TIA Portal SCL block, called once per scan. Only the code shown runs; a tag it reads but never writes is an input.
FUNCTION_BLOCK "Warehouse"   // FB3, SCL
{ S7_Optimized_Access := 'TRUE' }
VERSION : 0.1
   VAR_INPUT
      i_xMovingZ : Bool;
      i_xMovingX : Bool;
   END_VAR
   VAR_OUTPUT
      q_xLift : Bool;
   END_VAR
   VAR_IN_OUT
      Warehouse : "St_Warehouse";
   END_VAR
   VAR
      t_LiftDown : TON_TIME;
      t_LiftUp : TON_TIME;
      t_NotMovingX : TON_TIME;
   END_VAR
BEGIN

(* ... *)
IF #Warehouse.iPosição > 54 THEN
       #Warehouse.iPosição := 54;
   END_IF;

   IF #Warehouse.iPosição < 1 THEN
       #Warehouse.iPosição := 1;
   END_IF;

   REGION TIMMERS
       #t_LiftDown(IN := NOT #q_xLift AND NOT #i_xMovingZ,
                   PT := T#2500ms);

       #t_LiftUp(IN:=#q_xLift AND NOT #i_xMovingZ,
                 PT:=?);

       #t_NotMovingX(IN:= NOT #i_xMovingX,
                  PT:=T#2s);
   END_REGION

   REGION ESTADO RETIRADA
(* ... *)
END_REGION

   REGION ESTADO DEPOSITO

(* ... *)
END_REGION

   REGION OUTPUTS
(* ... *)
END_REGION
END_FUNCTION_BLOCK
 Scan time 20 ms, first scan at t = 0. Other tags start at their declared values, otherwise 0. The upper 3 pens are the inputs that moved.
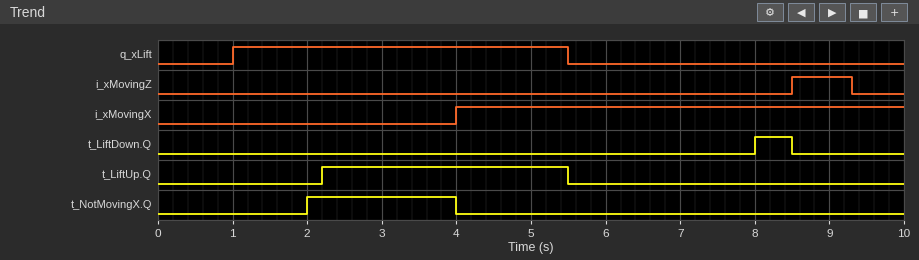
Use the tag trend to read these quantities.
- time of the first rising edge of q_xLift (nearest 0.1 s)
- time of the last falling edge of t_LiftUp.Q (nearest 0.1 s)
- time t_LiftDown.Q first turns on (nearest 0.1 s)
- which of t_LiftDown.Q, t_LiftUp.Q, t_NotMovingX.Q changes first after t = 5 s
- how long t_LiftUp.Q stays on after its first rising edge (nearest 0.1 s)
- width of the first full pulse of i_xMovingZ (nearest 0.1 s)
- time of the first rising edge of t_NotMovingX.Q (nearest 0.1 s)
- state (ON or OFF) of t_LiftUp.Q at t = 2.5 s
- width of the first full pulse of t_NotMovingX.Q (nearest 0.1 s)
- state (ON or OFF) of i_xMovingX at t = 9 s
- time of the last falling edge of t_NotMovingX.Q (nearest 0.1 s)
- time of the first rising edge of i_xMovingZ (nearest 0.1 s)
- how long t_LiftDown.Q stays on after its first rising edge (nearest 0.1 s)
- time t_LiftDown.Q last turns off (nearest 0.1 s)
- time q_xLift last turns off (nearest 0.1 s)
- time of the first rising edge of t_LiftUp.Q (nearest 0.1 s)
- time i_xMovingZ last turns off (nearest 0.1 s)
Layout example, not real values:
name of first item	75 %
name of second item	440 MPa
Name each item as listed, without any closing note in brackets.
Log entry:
time of the first rising edge of q_xLift	1.0 s
time of the last falling edge of t_LiftUp.Q	5.5 s
time t_LiftDown.Q first turns on	8.0 s
which of t_LiftDown.Q, t_LiftUp.Q, t_NotMovingX.Q changes first after t = 5 s	t_LiftUp.Q
how long t_LiftUp.Q stays on after its first rising edge	3.3 s
width of the first full pulse of i_xMovingZ	0.8 s
time of the first rising edge of t_NotMovingX.Q	2.0 s
state (ON or OFF) of t_LiftUp.Q at t = 2.5 s	ON
width of the first full pulse of t_NotMovingX.Q	2.0 s
state (ON or OFF) of i_xMovingX at t = 9 s	ON
time of the last falling edge of t_NotMovingX.Q	4.0 s
time of the first rising edge of i_xMovingZ	8.5 s
how long t_LiftDown.Q stays on after its first rising edge	0.5 s
time t_LiftDown.Q last turns off	8.5 s
time q_xLift last turns off	5.5 s
time of the first rising edge of t_LiftUp.Q	2.2 s
time i_xMovingZ last turns off	9.3 s
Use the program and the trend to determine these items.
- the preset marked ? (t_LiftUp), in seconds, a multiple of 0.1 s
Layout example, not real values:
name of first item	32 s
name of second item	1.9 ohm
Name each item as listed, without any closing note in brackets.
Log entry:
the preset marked ? (t_LiftUp), in seconds, a multiple of 0.1 s	1.2 s
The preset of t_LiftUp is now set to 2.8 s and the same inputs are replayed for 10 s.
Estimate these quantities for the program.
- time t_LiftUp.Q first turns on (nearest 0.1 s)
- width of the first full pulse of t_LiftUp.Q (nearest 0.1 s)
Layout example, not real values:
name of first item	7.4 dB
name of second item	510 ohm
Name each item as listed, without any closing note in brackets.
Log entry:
time t_LiftUp.Q first turns on	3.8 s
width of the first full pulse of t_LiftUp.Q	1.7 s
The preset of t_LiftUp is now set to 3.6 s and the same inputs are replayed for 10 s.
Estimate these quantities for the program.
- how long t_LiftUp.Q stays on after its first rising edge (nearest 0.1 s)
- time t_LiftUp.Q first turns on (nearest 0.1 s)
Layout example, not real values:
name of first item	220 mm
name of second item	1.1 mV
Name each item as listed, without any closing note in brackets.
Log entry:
how long t_LiftUp.Q stays on after its first rising edge	0.9 s
time t_LiftUp.Q first turns on	4.6 s
